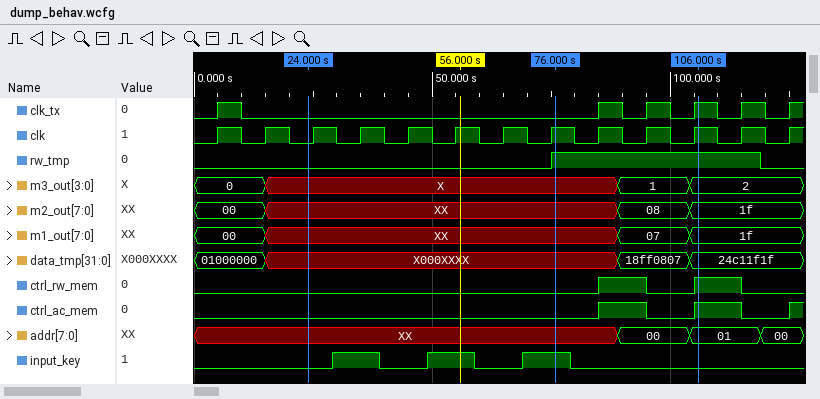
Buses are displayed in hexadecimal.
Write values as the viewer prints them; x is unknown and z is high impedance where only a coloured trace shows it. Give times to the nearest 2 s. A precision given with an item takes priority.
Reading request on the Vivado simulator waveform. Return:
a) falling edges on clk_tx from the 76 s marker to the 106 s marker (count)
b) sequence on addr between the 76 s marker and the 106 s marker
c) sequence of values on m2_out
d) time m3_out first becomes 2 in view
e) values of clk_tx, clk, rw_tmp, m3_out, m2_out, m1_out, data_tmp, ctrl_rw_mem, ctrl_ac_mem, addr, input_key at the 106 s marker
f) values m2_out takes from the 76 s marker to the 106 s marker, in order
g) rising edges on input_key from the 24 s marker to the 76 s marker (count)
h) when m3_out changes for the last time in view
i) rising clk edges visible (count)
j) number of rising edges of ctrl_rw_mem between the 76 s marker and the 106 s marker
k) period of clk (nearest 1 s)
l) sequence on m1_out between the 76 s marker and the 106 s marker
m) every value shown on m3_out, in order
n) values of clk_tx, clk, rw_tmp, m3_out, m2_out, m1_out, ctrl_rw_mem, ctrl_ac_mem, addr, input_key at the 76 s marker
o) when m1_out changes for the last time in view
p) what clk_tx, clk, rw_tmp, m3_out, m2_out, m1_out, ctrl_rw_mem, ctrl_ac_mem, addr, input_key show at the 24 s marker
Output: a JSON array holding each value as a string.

["2", "XX, 00, 01", "00, XX, 08, 1f", "104 s", "clk_tx=1, clk=1, rw_tmp=1, m3_out=2, m2_out=1f, m1_out=1f, data_tmp=24c11f1f, ctrl_rw_mem=1, ctrl_ac_mem=1, addr=01, input_key=0", "XX, 08, 1f", "3", "104 s", "13", "2", "10 s", "XX, 07, 1f", "0, X, 1, 2", "clk_tx=0, clk=1, rw_tmp=1, m3_out=X, m2_out=XX, m1_out=XX, ctrl_rw_mem=0, ctrl_ac_mem=0, addr=XX, input_key=1", "104 s", "clk_tx=0, clk=0, rw_tmp=0, m3_out=X, m2_out=XX, m1_out=XX, ctrl_rw_mem=0, ctrl_ac_mem=0, addr=XX, input_key=0"]
